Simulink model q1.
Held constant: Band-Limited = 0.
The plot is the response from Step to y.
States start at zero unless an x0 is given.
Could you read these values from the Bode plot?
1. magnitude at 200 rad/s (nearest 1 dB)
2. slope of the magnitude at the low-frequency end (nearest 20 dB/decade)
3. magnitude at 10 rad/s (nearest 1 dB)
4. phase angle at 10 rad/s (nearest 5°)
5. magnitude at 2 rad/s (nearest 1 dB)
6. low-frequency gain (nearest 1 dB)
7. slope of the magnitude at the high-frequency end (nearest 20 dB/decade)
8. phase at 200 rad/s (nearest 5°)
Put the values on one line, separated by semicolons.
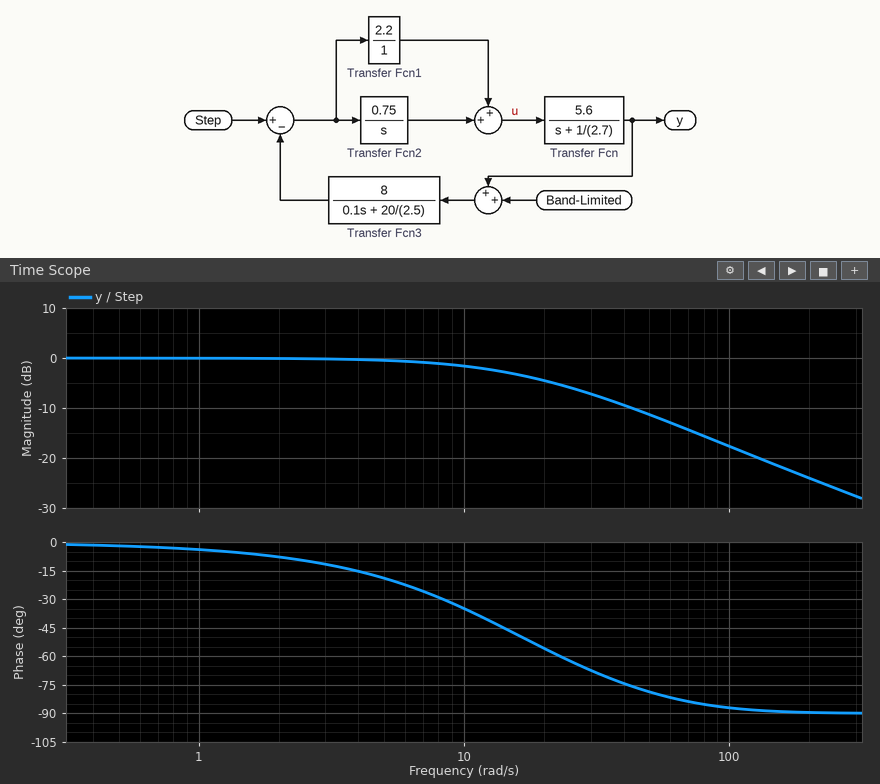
-24 dB; 0 dB/decade; -2 dB; -35°; 0 dB; 0 dB; -20 dB/decade; -90°
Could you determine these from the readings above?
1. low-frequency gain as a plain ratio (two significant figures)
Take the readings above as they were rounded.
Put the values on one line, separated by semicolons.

1.0
